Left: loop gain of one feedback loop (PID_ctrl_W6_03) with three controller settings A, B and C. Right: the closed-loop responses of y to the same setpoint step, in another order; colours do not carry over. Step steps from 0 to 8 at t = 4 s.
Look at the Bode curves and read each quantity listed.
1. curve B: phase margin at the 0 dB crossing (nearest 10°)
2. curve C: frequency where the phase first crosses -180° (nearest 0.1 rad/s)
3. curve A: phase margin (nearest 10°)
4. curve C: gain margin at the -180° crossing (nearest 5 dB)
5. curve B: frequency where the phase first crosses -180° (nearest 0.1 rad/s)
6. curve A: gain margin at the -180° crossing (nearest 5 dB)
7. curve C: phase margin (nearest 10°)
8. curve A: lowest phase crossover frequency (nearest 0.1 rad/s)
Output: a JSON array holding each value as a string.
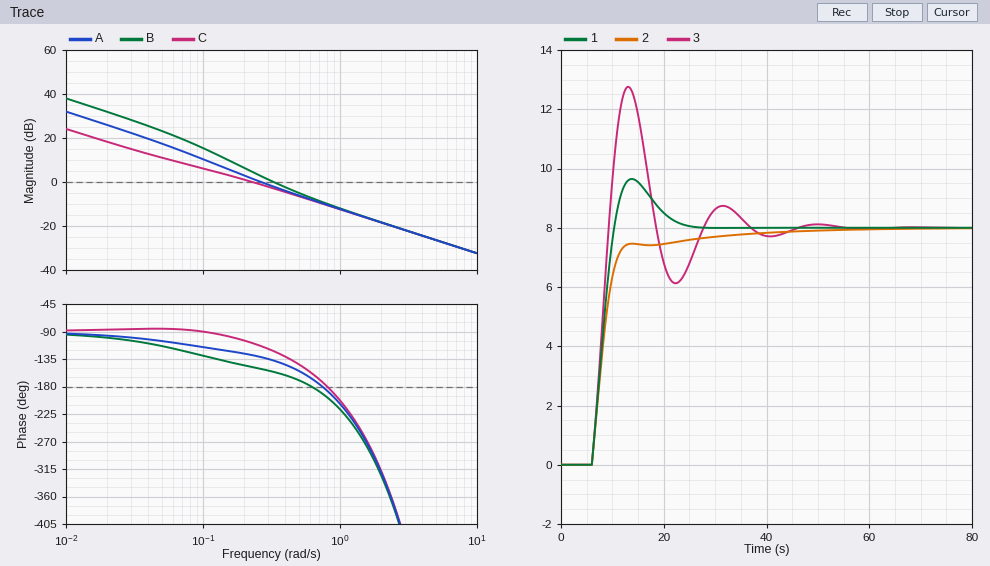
["20°", "0.8 rad/s", "50°", "10 dB", "0.6 rad/s", "10 dB", "70°", "0.7 rad/s"]
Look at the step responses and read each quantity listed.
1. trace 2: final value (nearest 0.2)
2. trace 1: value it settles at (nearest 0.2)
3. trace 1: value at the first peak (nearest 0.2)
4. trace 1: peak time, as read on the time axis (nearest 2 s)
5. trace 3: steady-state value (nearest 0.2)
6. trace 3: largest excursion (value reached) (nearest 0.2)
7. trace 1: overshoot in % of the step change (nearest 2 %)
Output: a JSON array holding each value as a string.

["8.0", "8.0", "9.6", "14 s", "8.0", "12.8", "20 %"]
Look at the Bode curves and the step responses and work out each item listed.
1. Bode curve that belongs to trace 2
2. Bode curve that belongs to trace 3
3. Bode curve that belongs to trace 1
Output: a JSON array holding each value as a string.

["C", "B", "A"]
